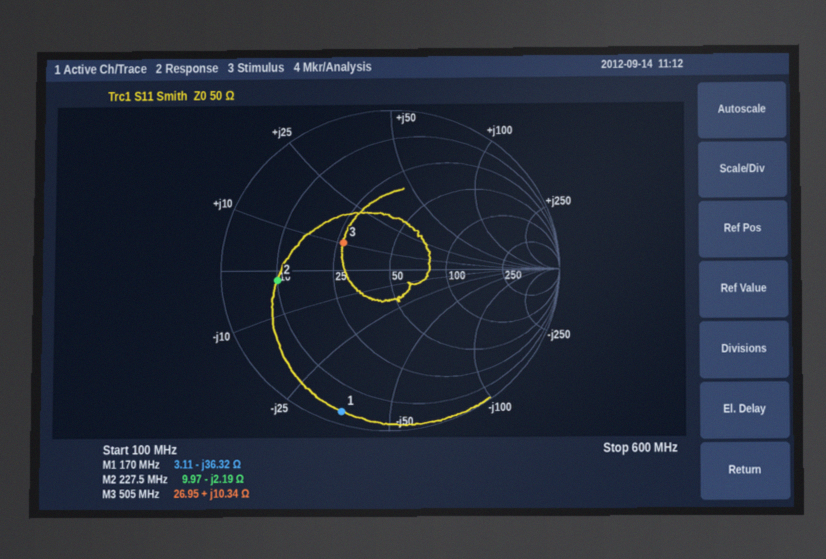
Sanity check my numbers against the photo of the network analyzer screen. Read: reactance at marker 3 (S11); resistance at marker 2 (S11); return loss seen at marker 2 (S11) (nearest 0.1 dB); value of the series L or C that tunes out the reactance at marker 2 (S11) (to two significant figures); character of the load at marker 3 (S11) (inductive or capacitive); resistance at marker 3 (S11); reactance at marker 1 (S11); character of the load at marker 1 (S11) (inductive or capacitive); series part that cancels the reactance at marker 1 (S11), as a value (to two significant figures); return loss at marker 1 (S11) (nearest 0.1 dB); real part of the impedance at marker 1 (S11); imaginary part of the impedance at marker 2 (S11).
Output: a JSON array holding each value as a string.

["+10.34 Ω", "9.97 Ω", "3.5 dB", "1.5 nH", "inductive", "26.95 Ω", "-36.32 Ω", "capacitive", "34 nH", "0.7 dB", "3.11 Ω", "-2.19 Ω"]
